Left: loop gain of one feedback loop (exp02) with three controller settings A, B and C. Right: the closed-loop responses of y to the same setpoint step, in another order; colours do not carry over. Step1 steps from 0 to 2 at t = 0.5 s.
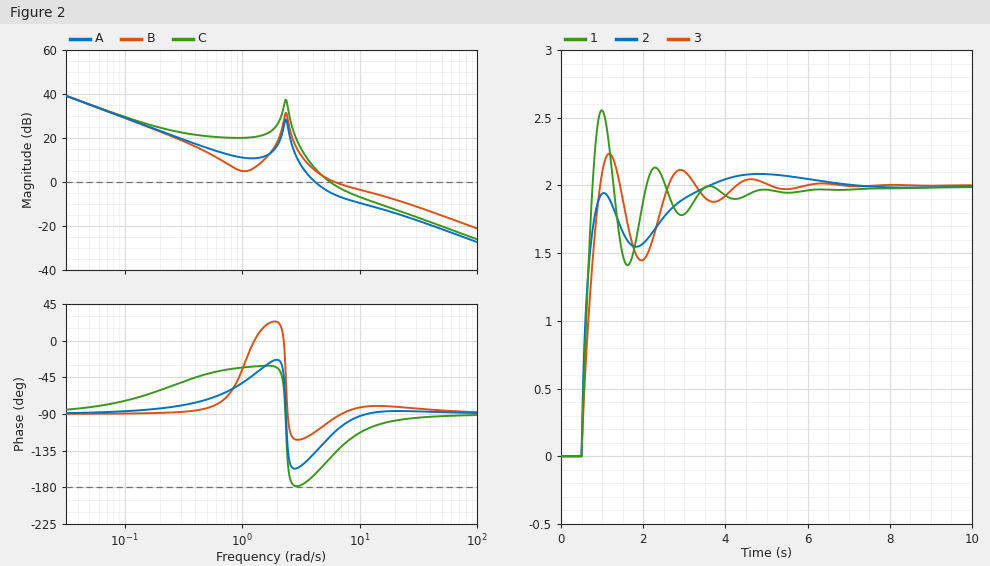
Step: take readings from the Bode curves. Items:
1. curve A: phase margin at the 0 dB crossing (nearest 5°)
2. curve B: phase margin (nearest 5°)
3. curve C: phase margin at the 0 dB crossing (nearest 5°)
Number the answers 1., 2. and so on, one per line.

1. 45°
2. 85°
3. 35°
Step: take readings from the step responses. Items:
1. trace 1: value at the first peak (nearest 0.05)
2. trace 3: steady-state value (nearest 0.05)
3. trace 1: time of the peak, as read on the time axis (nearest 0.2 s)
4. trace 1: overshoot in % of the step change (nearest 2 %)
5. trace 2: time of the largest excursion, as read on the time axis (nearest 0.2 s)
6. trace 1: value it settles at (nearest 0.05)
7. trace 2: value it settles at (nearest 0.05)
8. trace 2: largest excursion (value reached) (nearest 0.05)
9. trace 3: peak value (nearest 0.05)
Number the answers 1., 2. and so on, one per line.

1. 2.55
2. 2.00
3. 1.0 s
4. 28 %
5. 4.8 s
6. 2.00
7. 2.00
8. 2.10
9. 2.25
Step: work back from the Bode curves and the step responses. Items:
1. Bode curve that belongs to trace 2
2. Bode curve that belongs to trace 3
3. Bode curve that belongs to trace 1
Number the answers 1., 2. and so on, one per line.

1. B
2. A
3. C
